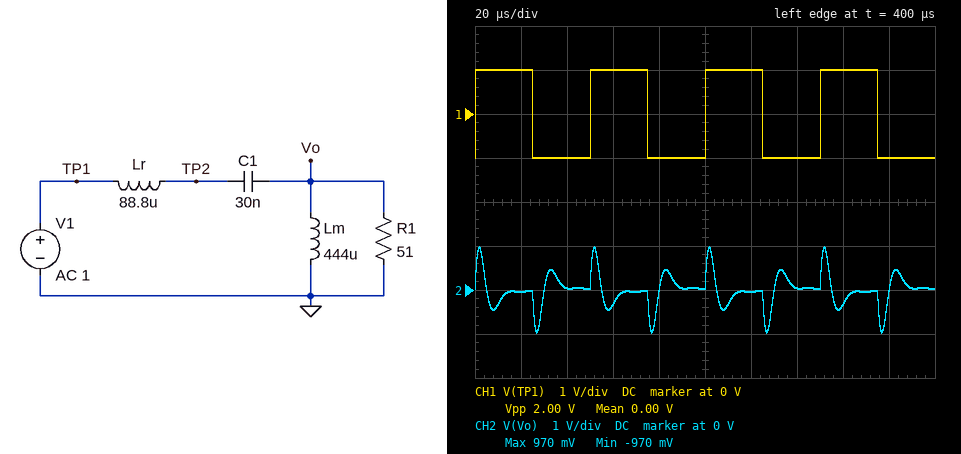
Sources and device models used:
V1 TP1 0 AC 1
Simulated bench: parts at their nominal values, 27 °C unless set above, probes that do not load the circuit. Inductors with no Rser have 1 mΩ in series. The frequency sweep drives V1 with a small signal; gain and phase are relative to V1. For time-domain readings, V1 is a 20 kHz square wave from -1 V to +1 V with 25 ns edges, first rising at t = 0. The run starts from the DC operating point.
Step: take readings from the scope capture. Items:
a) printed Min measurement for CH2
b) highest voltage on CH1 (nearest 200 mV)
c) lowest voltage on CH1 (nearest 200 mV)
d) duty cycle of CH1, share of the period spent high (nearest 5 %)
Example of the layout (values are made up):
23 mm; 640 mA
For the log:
-970 mV; 1.0 V; -1.0 V; 50 %
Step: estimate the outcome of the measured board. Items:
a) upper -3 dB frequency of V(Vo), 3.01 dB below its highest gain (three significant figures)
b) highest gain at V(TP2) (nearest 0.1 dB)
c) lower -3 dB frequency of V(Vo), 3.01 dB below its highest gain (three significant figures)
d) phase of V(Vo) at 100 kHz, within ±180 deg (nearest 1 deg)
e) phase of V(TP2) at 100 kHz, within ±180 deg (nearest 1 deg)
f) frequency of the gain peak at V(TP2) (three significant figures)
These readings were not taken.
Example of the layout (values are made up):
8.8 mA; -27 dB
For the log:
143 kHz; 3.5 dB; 55.8 kHz; -3 deg; -55 deg; 75.1 kHz
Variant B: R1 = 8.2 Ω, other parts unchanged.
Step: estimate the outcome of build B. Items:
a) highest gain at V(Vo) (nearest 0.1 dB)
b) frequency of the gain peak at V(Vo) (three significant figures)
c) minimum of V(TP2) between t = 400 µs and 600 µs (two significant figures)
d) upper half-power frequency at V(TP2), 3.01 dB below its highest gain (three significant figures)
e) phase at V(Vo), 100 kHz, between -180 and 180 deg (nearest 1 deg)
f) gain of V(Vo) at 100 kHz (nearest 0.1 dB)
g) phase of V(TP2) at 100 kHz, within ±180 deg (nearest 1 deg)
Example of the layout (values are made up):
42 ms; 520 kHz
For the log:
0 dB; 97.3 kHz; -3.1 V; 104 kHz; -18 deg; -0.5 dB; -101 deg
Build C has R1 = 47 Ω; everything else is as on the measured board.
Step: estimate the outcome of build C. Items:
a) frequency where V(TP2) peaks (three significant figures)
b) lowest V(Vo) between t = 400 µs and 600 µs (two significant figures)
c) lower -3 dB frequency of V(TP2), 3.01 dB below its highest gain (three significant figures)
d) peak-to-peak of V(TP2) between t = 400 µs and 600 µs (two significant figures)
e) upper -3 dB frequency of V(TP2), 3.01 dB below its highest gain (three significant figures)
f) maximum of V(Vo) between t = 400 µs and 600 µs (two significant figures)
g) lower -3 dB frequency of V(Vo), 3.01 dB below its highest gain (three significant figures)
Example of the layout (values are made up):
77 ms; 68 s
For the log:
77.9 kHz; -930 mV; 28.5 kHz; 3.3 V; 119 kHz; 930 mV; 58.6 kHz
